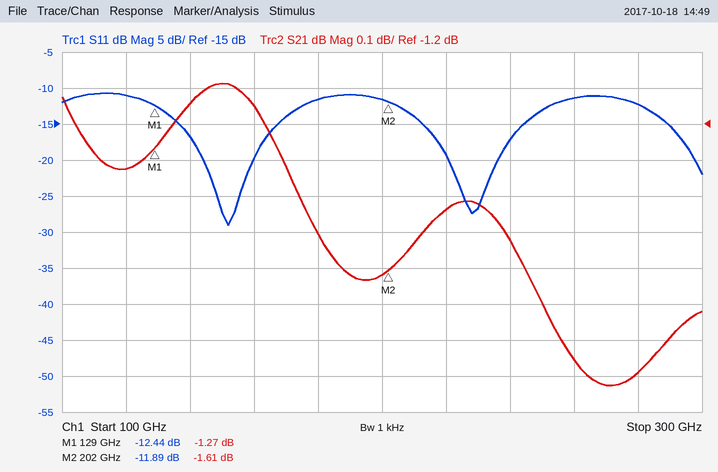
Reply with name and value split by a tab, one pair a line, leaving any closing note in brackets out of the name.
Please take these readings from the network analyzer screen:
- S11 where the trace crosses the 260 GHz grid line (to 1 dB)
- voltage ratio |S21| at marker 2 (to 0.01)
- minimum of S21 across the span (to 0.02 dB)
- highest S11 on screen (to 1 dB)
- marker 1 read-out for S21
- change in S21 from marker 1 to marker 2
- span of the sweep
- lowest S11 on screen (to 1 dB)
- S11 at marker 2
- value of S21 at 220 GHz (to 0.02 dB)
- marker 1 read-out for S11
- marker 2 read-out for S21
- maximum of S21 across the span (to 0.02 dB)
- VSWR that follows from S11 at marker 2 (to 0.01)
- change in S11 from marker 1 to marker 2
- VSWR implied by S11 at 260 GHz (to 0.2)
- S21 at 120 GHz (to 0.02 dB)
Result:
S11 where the trace crosses the 260 GHz grid line	-11 dB
voltage ratio |S21| at marker 2	0.83
minimum of S21 across the span	-1.92 dB
highest S11 on screen	-11 dB
marker 1 read-out for S21	-1.27 dB
change in S21 from marker 1 to marker 2	-0.34 dB
span of the sweep	200 GHz
lowest S11 on screen	-29 dB
S11 at marker 2	-11.89 dB
value of S21 at 220 GHz	-1.44 dB
marker 1 read-out for S11	-12.44 dB
marker 2 read-out for S21	-1.61 dB
maximum of S21 across the span	-1.08 dB
VSWR that follows from S11 at marker 2	1.68
change in S11 from marker 1 to marker 2	0.55 dB
VSWR implied by S11 at 260 GHz	1.8
S21 at 120 GHz	-1.32 dB
